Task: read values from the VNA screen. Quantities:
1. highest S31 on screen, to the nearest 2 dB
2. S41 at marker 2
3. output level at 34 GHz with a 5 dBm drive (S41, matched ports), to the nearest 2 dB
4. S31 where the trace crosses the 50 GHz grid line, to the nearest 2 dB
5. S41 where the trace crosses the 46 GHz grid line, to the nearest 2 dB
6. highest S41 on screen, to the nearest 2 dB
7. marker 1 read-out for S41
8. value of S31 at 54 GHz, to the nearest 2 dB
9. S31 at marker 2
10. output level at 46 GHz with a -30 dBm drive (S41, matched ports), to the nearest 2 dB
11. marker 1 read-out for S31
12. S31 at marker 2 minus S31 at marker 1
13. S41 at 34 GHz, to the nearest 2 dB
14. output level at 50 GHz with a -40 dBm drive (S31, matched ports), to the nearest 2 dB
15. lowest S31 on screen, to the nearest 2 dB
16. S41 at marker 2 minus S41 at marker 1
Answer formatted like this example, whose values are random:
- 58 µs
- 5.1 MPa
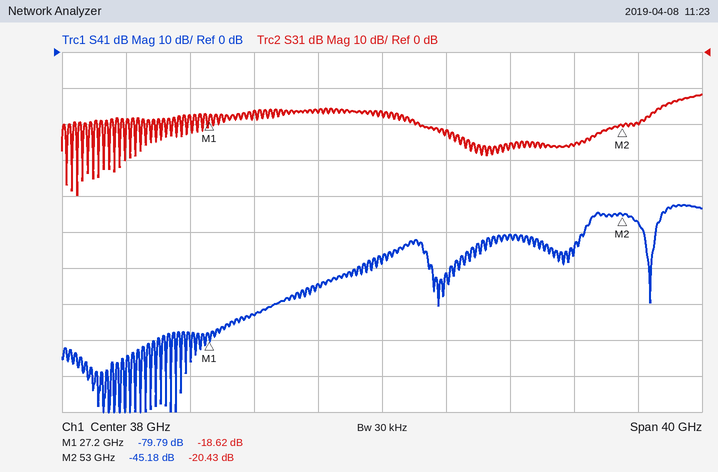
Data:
- -12 dB
- -45.18 dB
- -60 dBm
- -26 dB
- -50 dB
- -42 dB
- -79.79 dB
- -20 dB
- -20.43 dB
- -80 dBm
- -18.62 dB
- -1.81 dB
- -64 dB
- -66 dBm
- -40 dB
- 34.61 dB
